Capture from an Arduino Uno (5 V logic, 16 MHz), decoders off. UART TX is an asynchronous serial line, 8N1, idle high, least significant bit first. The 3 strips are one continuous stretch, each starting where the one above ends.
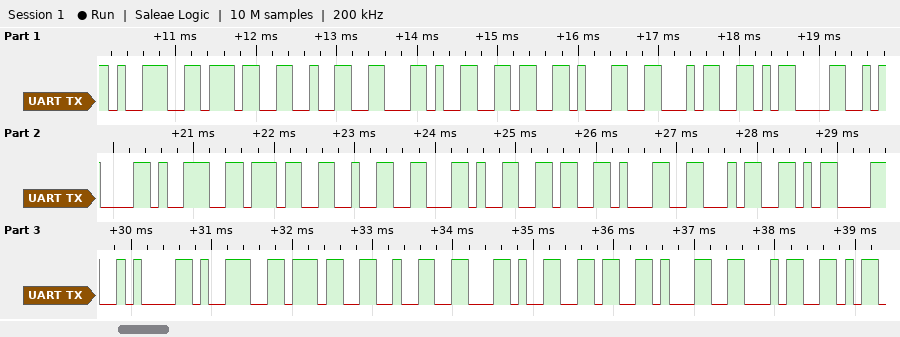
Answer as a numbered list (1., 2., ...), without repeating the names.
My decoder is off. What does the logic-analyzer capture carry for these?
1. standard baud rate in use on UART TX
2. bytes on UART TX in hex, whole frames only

1. 9600 baud
2. 39 37 32 2C 36 31 34 0D 0A 39 37 32 2C 36 31 34 0D 0A 39 37 32 2C 36 31 34
